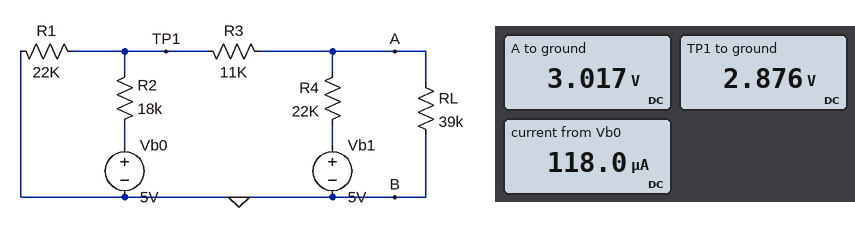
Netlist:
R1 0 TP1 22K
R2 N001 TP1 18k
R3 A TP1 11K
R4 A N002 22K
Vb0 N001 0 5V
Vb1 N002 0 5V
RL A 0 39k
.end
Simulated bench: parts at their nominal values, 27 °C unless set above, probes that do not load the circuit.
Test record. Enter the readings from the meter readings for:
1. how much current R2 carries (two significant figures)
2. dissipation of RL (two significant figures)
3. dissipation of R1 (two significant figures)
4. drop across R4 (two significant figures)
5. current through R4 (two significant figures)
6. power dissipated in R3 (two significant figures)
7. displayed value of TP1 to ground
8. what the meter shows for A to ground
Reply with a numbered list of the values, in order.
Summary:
1. 120 µA
2. 230 µW
3. 380 µW
4. 2.0 V
5. 90 µA
6. 1.8 µW
7. 2.876 V
8. 3.017 V
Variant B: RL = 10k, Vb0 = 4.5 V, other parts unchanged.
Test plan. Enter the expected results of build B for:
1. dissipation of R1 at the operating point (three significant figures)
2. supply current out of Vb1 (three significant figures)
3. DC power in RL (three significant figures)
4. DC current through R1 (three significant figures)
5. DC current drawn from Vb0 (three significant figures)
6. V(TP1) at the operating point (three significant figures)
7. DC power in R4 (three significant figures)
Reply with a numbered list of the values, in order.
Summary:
1. 210 µW
2. 146 µA
3. 320 µW
4. 97.7 µA
5. 131 µA
6. 2.15 V
7. 469 µW
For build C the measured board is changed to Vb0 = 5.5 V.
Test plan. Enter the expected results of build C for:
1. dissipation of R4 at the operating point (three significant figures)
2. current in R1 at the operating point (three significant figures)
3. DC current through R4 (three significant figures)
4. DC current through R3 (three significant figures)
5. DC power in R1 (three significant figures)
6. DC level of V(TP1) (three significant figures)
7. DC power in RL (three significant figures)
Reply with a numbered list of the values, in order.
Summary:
1. 159 µW
2. 140 µA
3. 85.1 µA
4. 4.91 µA
5. 429 µW
6. 3.07 V
7. 251 µW
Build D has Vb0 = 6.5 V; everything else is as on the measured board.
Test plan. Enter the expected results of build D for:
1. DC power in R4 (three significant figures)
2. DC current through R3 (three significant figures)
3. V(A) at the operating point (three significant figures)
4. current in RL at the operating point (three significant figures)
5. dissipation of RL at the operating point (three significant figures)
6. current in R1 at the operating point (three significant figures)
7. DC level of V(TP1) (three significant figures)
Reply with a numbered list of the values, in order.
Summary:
1. 124 µW
2. 10.8 µA
3. 3.35 V
4. 85.9 µA
5. 288 µW
6. 158 µA
7. 3.47 V
